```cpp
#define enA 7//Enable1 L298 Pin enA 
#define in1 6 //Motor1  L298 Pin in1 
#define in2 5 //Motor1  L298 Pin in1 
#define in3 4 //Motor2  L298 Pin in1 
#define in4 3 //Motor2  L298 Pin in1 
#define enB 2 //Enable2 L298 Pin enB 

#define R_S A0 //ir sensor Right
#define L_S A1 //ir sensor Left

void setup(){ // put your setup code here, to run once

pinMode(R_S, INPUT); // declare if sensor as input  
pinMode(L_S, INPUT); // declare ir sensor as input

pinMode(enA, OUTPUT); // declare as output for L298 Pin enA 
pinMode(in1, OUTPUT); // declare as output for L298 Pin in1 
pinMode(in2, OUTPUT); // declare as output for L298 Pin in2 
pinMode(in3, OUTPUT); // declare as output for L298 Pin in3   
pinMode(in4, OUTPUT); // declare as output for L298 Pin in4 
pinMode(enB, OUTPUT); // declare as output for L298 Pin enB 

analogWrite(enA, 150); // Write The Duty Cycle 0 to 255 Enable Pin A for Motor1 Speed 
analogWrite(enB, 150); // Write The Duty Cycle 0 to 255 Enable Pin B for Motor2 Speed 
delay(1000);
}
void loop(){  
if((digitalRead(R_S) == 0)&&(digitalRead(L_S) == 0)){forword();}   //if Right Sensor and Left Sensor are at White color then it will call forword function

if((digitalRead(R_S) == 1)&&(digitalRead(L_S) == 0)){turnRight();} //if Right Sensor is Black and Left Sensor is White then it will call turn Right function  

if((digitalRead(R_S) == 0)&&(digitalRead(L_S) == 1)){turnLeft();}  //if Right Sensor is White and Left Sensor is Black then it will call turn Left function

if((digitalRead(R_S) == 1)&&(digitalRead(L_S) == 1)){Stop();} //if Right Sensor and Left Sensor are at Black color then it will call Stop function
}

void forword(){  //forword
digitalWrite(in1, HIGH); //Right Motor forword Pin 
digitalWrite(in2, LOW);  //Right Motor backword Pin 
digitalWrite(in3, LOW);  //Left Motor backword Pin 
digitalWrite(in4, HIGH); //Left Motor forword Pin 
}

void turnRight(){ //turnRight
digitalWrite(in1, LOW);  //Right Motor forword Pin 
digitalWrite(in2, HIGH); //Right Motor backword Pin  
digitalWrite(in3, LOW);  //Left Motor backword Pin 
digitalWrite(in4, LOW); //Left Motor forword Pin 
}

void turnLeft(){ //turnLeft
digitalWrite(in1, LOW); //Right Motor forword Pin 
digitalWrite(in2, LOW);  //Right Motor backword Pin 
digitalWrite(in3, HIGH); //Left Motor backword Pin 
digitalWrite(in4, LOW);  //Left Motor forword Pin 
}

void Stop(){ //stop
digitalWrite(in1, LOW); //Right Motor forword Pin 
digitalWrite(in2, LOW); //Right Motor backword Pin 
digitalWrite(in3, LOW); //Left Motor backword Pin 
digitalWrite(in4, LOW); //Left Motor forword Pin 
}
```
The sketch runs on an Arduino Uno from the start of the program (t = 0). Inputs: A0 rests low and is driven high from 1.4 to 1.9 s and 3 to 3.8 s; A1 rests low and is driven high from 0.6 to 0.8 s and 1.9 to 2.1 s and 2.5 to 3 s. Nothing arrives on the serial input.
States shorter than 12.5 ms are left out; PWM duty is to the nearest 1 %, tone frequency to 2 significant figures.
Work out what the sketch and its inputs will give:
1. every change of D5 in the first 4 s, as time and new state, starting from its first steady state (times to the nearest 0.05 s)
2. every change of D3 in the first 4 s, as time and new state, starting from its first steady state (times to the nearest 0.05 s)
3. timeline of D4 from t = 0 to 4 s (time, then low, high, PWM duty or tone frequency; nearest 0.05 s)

0 s low; 1.4 s high; 1.9 s low; 3 s high; 3.8 s low
0 s low; 1 s high; 1.4 s low; 2.1 s high; 2.5 s low; 3.8 s high
0 s low; 1.9 s high; 2.1 s low; 2.5 s high; 3 s low
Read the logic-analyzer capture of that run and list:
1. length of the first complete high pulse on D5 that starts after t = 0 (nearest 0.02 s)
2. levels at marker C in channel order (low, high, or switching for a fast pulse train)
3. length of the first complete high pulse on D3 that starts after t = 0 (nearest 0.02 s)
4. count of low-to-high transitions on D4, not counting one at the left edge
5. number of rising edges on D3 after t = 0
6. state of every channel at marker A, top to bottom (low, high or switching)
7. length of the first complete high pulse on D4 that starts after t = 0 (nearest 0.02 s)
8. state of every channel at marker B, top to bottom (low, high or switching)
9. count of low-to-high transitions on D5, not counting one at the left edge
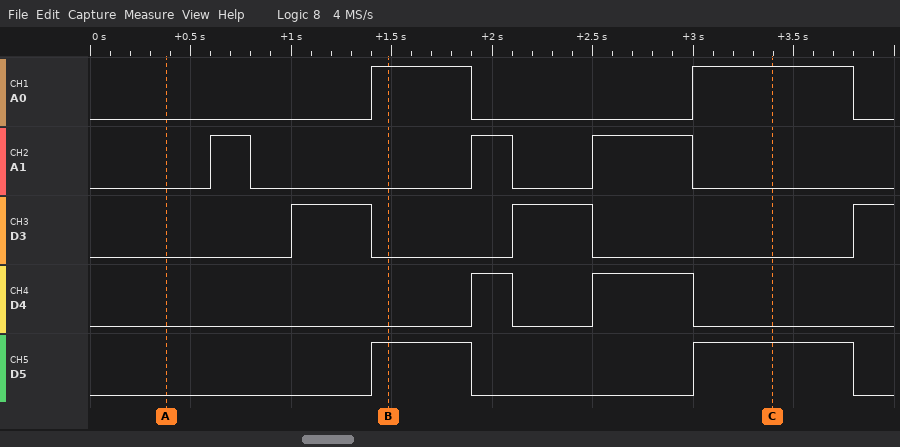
0.50 s
A0 high, A1 low, D3 low, D4 low, D5 high
0.40 s
2
3
A0 low, A1 low, D3 low, D4 low, D5 low
0.20 s
A0 high, A1 low, D3 low, D4 low, D5 high
2
